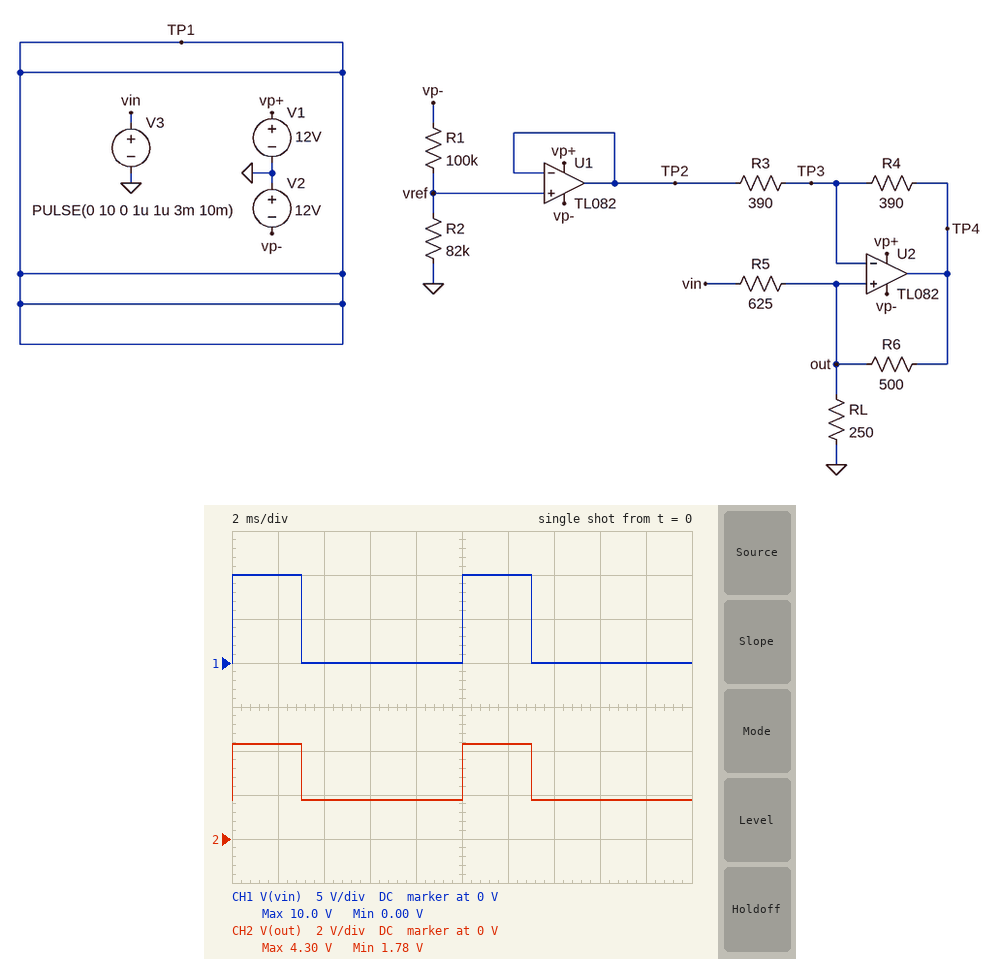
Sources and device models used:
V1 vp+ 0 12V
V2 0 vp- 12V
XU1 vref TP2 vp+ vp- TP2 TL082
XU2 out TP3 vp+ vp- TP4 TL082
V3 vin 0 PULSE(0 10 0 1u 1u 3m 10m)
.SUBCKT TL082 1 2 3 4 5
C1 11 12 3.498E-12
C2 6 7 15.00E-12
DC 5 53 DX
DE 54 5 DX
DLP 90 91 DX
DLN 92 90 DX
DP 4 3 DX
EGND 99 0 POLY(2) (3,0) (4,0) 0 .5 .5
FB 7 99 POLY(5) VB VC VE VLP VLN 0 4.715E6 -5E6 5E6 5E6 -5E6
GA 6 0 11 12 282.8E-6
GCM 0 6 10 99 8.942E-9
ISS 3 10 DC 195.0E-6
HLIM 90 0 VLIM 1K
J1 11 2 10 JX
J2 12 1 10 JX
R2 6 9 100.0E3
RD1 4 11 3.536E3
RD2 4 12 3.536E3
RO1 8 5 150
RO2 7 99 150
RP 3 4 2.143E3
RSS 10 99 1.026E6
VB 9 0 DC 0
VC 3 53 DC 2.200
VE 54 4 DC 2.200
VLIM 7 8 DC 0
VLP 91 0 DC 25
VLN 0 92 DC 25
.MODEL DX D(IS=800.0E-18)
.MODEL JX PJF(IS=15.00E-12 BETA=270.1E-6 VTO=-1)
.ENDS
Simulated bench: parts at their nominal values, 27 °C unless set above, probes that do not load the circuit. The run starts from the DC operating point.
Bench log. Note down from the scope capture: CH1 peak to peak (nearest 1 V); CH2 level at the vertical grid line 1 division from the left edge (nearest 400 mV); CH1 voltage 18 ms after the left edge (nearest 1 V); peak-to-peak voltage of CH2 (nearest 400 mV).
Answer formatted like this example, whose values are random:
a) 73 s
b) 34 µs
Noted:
a) 10 V
b) 4.4 V
c) 0 V
d) 2.4 V
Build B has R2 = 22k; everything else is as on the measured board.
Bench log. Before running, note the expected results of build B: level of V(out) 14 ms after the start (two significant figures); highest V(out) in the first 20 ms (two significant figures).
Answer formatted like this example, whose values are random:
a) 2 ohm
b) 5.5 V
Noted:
a) 1.2 V
b) 4.7 V
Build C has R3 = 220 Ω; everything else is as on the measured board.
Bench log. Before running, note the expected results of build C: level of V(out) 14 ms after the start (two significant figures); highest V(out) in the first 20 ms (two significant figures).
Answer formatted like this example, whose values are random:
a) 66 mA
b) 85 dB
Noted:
a) 1.4 V
b) 3.9 V
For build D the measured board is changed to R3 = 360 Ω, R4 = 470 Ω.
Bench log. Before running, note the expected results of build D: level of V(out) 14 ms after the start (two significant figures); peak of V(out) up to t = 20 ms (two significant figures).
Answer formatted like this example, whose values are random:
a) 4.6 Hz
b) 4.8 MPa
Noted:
a) 1.9 V
b) 4.4 V
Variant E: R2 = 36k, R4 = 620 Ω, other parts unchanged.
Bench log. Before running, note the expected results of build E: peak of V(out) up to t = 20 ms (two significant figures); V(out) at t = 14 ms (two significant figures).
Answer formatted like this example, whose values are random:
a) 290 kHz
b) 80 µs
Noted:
a) 4.9 V
b) 2.4 V
